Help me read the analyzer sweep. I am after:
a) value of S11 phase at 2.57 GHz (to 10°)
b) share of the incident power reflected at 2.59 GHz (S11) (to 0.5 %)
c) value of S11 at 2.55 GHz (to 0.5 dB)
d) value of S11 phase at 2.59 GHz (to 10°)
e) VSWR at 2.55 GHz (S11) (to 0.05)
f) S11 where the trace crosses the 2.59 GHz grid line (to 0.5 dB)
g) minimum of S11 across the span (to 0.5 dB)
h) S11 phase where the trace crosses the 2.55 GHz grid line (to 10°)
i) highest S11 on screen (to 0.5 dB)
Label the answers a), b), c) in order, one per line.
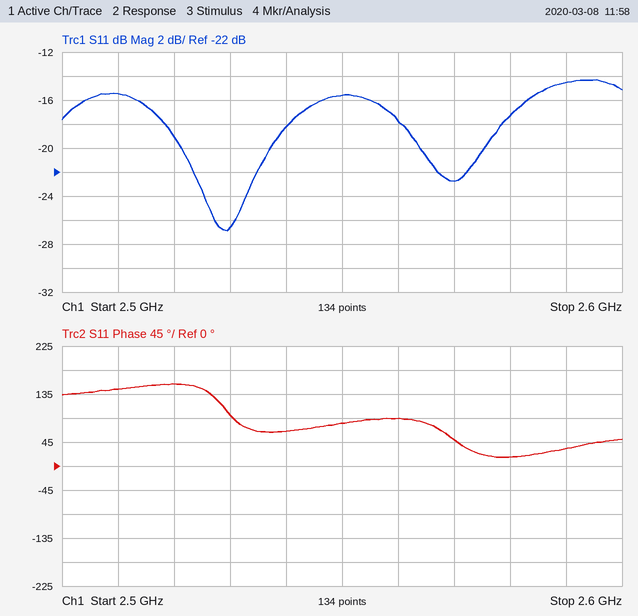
a) 50°
b) 3.5 %
c) -15.5 dB
d) 30°
e) 1.40
f) -14.5 dB
g) -27.0 dB
h) 80°
i) -14.5 dB
